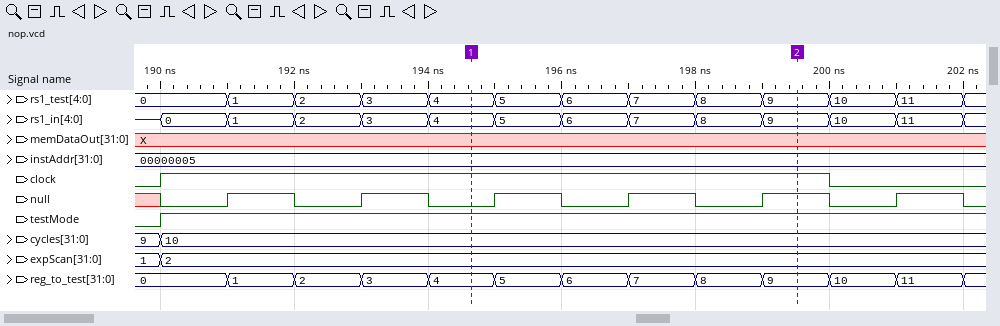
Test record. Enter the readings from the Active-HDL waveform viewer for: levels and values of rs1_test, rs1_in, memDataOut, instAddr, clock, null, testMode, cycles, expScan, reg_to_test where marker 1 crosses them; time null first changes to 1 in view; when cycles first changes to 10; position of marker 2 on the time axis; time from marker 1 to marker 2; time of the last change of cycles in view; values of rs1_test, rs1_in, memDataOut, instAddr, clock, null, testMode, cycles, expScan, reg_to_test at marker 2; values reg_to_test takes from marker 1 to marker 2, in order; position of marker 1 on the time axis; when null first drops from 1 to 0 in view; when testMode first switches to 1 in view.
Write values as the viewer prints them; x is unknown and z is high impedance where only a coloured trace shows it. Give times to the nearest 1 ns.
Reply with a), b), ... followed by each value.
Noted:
a) rs1_test=4, rs1_in=4, memDataOut=X, instAddr=00000005, clock=1, null=0, testMode=1, cycles=10, expScan=2, reg_to_test=4
b) 191 ns
c) 190 ns
d) 200 ns
e) 5 ns
f) 190 ns
g) rs1_test=9, rs1_in=9, memDataOut=X, instAddr=00000005, clock=1, null=1, testMode=1, cycles=10, expScan=2, reg_to_test=9
h) 4, 5, 6, 7, 8, 9
i) 195 ns
j) 192 ns
k) 190 ns
